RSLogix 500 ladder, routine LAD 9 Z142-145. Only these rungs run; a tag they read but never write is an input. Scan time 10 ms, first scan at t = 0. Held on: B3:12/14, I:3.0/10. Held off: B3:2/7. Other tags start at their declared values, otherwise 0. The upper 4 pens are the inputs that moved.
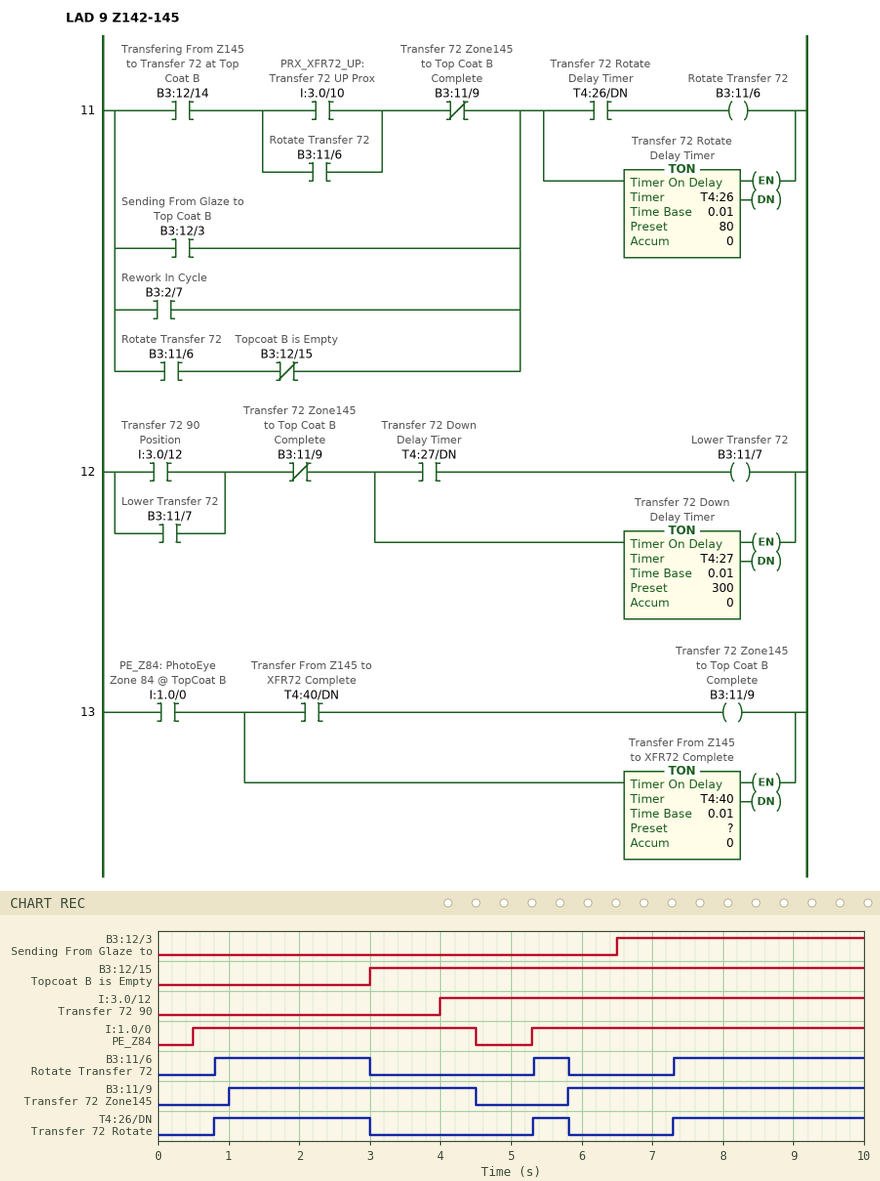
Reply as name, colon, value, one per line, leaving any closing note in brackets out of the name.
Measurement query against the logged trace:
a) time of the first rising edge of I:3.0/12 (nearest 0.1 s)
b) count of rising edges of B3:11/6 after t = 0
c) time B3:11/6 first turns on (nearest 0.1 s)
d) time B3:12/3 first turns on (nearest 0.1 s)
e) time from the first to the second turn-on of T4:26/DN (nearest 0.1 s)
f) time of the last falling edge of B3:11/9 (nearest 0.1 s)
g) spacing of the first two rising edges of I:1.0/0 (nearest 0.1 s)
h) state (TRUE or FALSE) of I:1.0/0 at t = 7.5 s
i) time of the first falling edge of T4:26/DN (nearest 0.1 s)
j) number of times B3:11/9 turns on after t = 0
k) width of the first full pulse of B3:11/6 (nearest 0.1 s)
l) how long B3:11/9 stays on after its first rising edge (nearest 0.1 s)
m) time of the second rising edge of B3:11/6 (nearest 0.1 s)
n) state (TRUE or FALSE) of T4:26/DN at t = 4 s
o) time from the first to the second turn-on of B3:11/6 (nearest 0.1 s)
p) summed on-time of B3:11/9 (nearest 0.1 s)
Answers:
time of the first rising edge of I:3.0/12: 4.0 s
count of rising edges of B3:11/6 after t = 0: 3
time B3:11/6 first turns on: 0.8 s
time B3:12/3 first turns on: 6.5 s
time from the first to the second turn-on of T4:26/DN: 4.5 s
time of the last falling edge of B3:11/9: 4.5 s
spacing of the first two rising edges of I:1.0/0: 4.8 s
state (TRUE or FALSE) of I:1.0/0 at t = 7.5 s: TRUE
time of the first falling edge of T4:26/DN: 3.0 s
number of times B3:11/9 turns on after t = 0: 2
width of the first full pulse of B3:11/6: 2.2 s
how long B3:11/9 stays on after its first rising edge: 3.5 s
time of the second rising edge of B3:11/6: 5.3 s
state (TRUE or FALSE) of T4:26/DN at t = 4 s: FALSE
time from the first to the second turn-on of B3:11/6: 4.5 s
summed on-time of B3:11/9: 7.7 s
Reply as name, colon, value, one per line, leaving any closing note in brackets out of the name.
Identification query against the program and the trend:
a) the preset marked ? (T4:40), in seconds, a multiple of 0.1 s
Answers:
the preset marked ? (T4:40), in seconds, a multiple of 0.1 s: 0.5 s
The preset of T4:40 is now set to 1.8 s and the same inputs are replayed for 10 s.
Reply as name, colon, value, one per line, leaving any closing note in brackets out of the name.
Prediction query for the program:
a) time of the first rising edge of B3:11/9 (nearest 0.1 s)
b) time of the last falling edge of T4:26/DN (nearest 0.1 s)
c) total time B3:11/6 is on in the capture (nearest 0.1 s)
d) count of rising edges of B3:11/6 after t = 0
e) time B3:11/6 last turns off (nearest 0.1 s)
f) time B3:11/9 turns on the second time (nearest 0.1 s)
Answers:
time of the first rising edge of B3:11/9: 2.3 s
time of the last falling edge of T4:26/DN: 3.0 s
total time B3:11/6 is on in the capture: 6.9 s
count of rising edges of B3:11/6 after t = 0: 2
time B3:11/6 last turns off: 3.0 s
time B3:11/9 turns on the second time: 7.1 s
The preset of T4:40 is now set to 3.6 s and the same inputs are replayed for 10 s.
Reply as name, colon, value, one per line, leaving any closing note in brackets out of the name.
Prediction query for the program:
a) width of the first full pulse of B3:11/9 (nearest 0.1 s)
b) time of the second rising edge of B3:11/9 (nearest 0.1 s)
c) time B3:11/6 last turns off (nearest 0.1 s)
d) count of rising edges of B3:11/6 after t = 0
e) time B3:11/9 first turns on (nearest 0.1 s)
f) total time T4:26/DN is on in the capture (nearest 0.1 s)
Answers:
width of the first full pulse of B3:11/9: 0.4 s
time of the second rising edge of B3:11/9: 8.9 s
time B3:11/6 last turns off: 4.1 s
count of rising edges of B3:11/6 after t = 0: 2
time B3:11/9 first turns on: 4.1 s
total time T4:26/DN is on in the capture: 8.0 s
